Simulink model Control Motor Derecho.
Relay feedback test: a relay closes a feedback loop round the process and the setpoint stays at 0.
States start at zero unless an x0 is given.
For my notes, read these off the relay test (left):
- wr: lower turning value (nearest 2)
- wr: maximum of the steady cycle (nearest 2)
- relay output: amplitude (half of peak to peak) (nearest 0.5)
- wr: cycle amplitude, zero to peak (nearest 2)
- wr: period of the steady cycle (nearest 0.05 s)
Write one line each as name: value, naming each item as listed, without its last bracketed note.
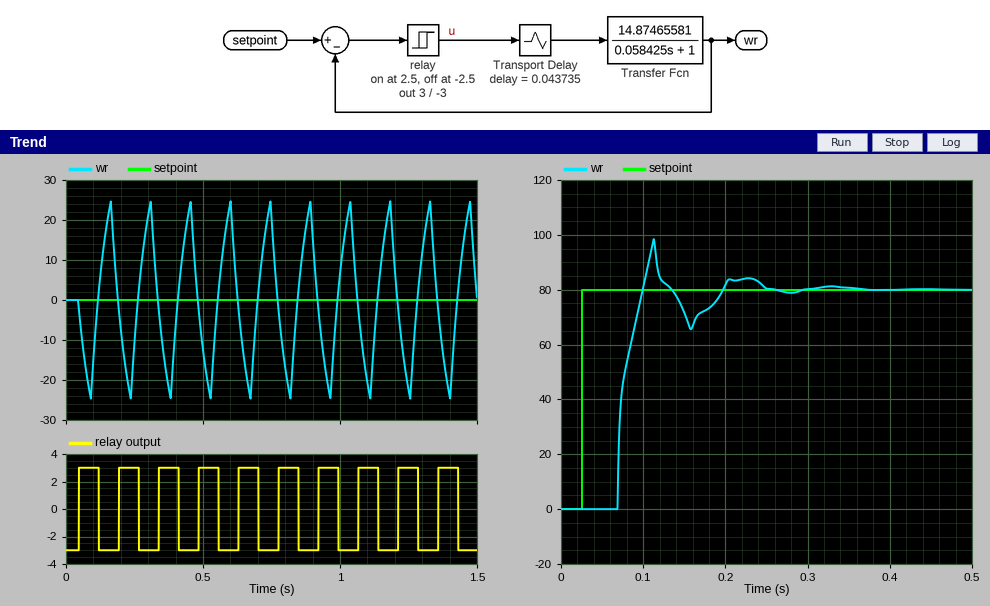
wr: lower turning value: -24
wr: maximum of the steady cycle: 24
relay output: amplitude (half of peak to peak): 3.0
wr: cycle amplitude, zero to peak: 24
wr: period of the steady cycle: 0.15 s
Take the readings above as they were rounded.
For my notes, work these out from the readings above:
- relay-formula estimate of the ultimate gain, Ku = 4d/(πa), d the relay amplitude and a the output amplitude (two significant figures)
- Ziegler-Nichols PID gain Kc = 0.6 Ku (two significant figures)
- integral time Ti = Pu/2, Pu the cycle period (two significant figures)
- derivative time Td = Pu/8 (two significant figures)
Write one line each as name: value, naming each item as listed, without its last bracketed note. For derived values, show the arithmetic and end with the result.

relay-formula estimate of the ultimate gain, Ku = 4d/(πa), d the relay amplitude and a the output amplitude: 4 × 3 / (π × 24) = 0.16
Ziegler-Nichols PID gain Kc = 0.6 Ku: 0.6 × 0.16 = 0.096
integral time Ti = Pu/2, Pu the cycle period: 0.15 / 2 = 0.075 s
derivative time Td = Pu/8: 0.15 / 8 = 0.019 s
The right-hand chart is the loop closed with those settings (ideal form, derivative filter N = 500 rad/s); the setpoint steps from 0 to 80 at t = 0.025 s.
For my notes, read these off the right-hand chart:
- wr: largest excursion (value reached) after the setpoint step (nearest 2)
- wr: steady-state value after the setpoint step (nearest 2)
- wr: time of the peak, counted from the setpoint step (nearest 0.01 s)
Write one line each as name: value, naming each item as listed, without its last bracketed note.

wr: largest excursion (value reached) after the setpoint step: 98
wr: steady-state value after the setpoint step: 80
wr: time of the peak, counted from the setpoint step: 0.09 s
